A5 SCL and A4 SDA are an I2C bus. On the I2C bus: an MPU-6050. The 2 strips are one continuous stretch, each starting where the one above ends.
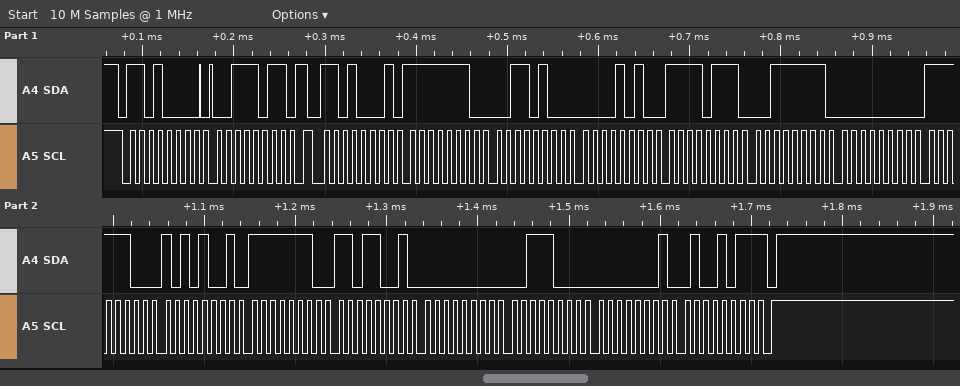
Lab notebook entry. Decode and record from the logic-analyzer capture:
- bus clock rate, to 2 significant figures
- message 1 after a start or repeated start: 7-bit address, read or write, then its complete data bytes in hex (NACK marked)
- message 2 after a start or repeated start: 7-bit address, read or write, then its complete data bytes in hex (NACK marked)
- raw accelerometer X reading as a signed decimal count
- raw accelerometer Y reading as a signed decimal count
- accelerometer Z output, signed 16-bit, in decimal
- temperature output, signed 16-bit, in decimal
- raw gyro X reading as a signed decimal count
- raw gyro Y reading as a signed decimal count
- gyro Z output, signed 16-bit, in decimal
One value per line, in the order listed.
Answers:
100 kHz
0x68 write: 3B
0x68 read: FE 34 0A F7 3F 00 FC A9 FE D9 00 38 01 4B NACK
-460
2807
16128
-855
-295
56
331
